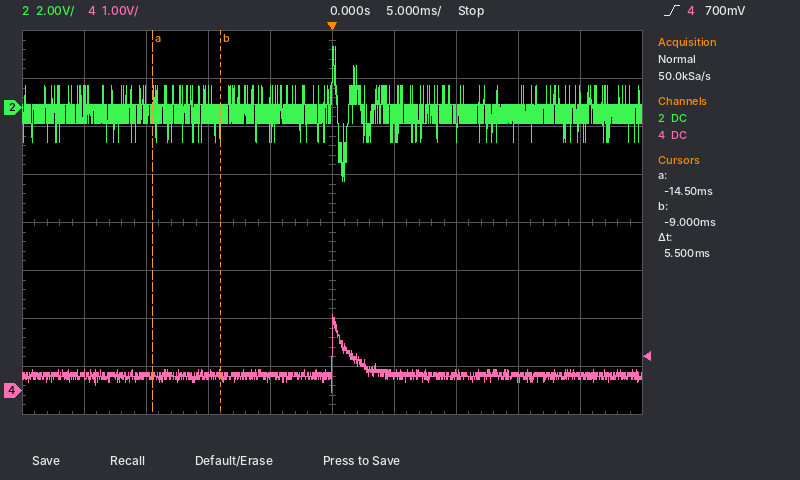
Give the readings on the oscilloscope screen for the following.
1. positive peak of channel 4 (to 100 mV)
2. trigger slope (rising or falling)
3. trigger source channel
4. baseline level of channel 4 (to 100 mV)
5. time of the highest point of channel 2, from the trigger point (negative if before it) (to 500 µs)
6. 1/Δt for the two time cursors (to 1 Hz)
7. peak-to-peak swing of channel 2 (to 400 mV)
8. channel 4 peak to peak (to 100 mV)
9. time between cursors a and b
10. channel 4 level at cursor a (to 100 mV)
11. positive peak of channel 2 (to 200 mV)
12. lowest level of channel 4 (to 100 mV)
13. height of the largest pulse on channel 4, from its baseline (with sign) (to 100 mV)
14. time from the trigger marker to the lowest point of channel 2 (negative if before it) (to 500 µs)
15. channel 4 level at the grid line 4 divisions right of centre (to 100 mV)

1.6 V
rising
channel 4
300 mV
0.0 ms
182 Hz
5.6 V
1.6 V
5.5 ms
300 mV
2.6 V
0.0 V
+1.3 V
+1.0 ms
300 mV
